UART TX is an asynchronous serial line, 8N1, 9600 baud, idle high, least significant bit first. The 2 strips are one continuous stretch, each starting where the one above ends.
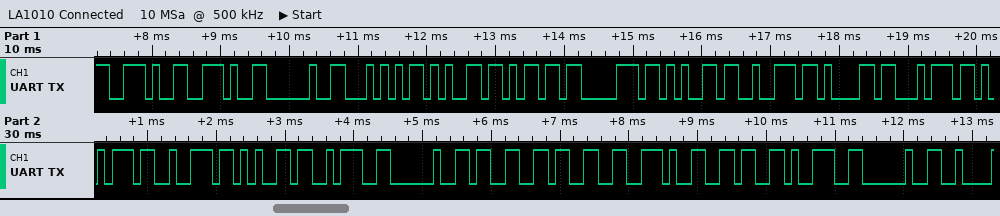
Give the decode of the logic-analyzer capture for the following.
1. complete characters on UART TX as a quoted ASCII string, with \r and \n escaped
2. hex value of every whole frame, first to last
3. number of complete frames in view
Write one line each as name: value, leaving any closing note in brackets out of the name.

complete characters on UART TX as a quoted ASCII string, with \r and \n escaped: ".. Temperature: 33.69 "
hex value of every whole frame, first to last: 2E 2E 20 54 65 6D 70 65 72 61 74 75 72 65 3A 20 33 33 2E 36 39 20
number of complete frames in view: 22
